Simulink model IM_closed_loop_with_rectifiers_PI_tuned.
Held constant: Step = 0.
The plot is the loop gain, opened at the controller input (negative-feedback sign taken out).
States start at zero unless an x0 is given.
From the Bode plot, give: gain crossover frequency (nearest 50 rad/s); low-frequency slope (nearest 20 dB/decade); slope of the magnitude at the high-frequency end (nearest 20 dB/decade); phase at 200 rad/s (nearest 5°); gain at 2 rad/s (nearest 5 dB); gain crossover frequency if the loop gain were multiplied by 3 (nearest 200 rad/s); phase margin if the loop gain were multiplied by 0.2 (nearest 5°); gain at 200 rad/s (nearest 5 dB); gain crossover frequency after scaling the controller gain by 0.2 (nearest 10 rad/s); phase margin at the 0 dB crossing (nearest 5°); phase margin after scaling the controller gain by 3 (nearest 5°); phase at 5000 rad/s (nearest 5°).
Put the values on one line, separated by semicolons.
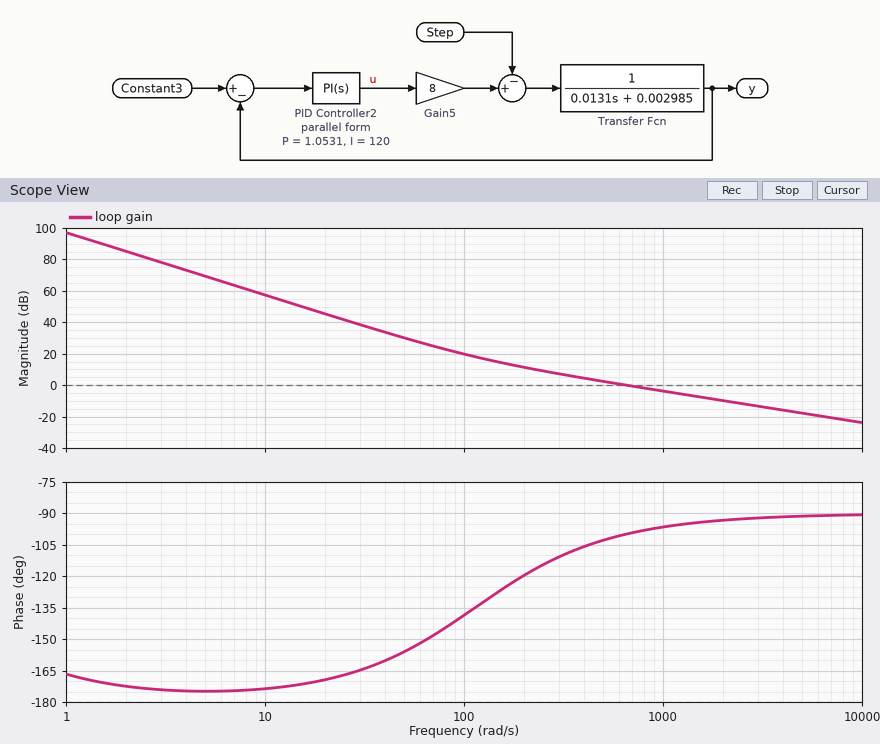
650 rad/s; -40 dB/decade; -20 dB/decade; -120°; 85 dB; 2000 rad/s; 55°; 10 dB; 160 rad/s; 80°; 85°; -90°
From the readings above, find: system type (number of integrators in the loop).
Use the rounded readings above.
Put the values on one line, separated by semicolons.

2
